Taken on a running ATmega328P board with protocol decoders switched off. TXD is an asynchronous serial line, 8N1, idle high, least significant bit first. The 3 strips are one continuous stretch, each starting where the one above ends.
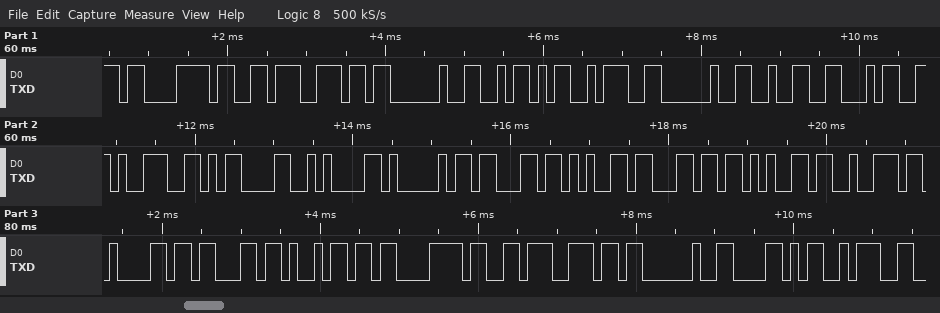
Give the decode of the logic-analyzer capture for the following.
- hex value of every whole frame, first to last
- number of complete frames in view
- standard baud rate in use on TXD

0xC3 0xB3 0x6E 0x20 0x5A 0x3A 0x20 0x32 0x34 0x39 0x0D 0x0A 0x41 0x63 0x65 0x6C 0x65 0x72 0x61 0x63 0x69 0xC3 0xB3 0x6E 0x20 0x58 0x3A
27
9600 baud
